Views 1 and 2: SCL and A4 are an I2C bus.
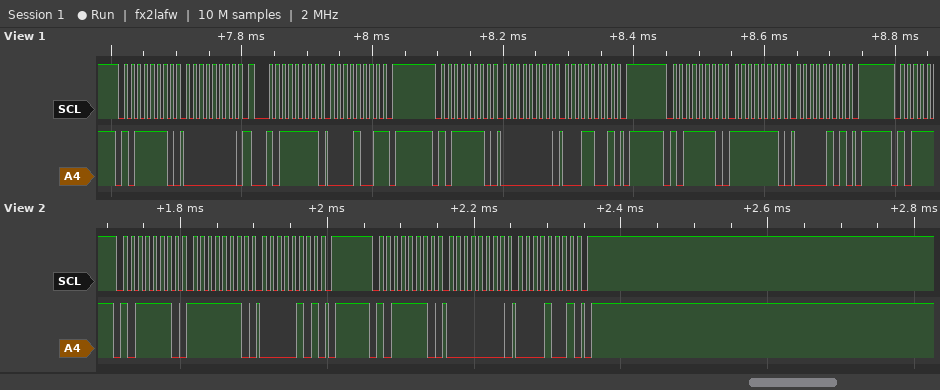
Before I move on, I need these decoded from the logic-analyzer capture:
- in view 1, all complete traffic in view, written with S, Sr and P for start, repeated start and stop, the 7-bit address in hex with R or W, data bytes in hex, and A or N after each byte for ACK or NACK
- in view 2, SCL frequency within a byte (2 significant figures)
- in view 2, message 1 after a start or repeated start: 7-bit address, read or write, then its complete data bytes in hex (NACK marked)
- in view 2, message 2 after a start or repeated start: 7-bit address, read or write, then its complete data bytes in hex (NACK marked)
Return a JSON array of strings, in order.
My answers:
["S 5FW A 00 A Sr 5FR A 09 N P S 5FW A 00 A 19 A P S 5FW A FE A 05 A P", "100 kHz", "0x5F write: FE 05", "0x5F write: 00 09"]
